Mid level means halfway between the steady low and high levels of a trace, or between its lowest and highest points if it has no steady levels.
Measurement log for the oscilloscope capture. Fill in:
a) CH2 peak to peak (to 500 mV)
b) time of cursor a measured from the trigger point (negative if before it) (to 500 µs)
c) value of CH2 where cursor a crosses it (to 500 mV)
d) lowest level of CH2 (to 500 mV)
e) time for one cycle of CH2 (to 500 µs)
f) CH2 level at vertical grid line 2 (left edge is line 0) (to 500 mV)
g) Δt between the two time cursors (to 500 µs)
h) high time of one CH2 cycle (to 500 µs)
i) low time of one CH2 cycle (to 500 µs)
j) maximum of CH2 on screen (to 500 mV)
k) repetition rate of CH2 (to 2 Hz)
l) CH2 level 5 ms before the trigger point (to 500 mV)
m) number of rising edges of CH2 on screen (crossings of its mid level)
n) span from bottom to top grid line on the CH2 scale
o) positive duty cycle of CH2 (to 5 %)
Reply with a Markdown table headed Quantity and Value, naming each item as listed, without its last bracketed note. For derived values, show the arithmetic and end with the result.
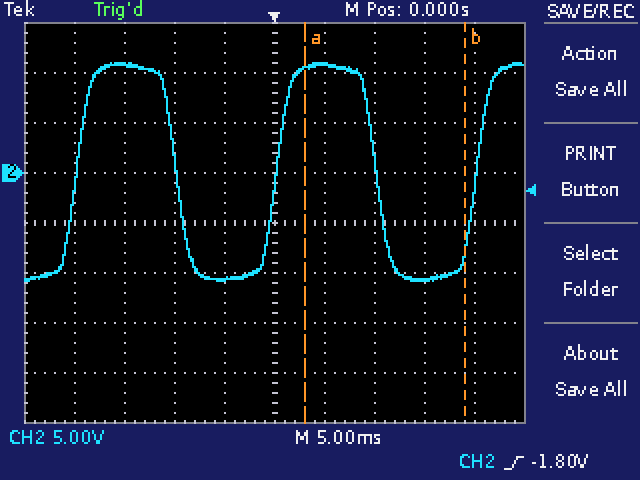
| Quantity | Value |
|---|---|
| CH2 peak to peak | 11.0 V − (-11.0 V) = 22.0 V |
| time of cursor a measured from the trigger point (negative if before it) | +3.0 ms |
| value of CH2 where cursor a crosses it | 10.5 V |
| lowest level of CH2 | -11.0 V |
| time for one cycle of CH2 | 20.0 ms |
| CH2 level at vertical grid line 2 (left edge is line 0) | 11.0 V |
| Δt between the two time cursors | 16.0 ms |
| high time of one CH2 cycle | 10.0 ms |
| low time of one CH2 cycle | 10.0 ms |
| maximum of CH2 on screen | 11.0 V |
| repetition rate of CH2 | 1 / 20.0 ms ≈ 50 Hz |
| CH2 level 5 ms before the trigger point | -10.5 V |
| number of rising edges of CH2 on screen | 3 |
| span from bottom to top grid line on the CH2 scale | 40 V |
| positive duty cycle of CH2 | 10.0 ms / 20.0 ms ≈ 50 % |
